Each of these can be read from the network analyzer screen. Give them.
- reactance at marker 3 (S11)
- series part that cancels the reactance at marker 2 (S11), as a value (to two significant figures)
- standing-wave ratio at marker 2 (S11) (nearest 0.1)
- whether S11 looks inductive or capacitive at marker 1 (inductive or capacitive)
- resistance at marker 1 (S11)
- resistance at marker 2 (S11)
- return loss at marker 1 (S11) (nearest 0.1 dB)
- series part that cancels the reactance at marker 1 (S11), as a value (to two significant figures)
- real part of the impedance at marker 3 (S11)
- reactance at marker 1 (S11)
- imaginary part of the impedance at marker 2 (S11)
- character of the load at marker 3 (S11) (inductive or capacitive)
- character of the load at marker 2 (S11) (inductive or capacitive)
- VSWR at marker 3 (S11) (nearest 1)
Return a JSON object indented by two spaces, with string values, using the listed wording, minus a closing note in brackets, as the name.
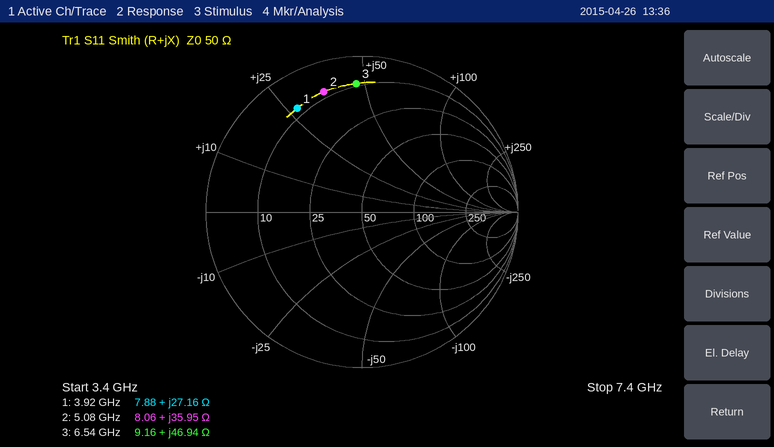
{
  "reactance at marker 3": "+46.94 Ω",
  "series part that cancels the reactance at marker 2 (S11), as a value": "870 fF",
  "standing-wave ratio at marker 2 (S11)": "9.5",
  "whether S11 looks inductive or capacitive at marker 1": "inductive",
  "resistance at marker 1": "7.88 Ω",
  "resistance at marker 2": "8.06 Ω",
  "return loss at marker 1 (S11)": "2.1 dB",
  "series part that cancels the reactance at marker 1 (S11), as a value": "1.5 pF",
  "real part of the impedance at marker 3": "9.16 Ω",
  "reactance at marker 1": "+27.16 Ω",
  "imaginary part of the impedance at marker 2": "+35.95 Ω",
  "character of the load at marker 3 (S11)": "inductive",
  "character of the load at marker 2 (S11)": "inductive",
  "VSWR at marker 3 (S11)": "10"
}
